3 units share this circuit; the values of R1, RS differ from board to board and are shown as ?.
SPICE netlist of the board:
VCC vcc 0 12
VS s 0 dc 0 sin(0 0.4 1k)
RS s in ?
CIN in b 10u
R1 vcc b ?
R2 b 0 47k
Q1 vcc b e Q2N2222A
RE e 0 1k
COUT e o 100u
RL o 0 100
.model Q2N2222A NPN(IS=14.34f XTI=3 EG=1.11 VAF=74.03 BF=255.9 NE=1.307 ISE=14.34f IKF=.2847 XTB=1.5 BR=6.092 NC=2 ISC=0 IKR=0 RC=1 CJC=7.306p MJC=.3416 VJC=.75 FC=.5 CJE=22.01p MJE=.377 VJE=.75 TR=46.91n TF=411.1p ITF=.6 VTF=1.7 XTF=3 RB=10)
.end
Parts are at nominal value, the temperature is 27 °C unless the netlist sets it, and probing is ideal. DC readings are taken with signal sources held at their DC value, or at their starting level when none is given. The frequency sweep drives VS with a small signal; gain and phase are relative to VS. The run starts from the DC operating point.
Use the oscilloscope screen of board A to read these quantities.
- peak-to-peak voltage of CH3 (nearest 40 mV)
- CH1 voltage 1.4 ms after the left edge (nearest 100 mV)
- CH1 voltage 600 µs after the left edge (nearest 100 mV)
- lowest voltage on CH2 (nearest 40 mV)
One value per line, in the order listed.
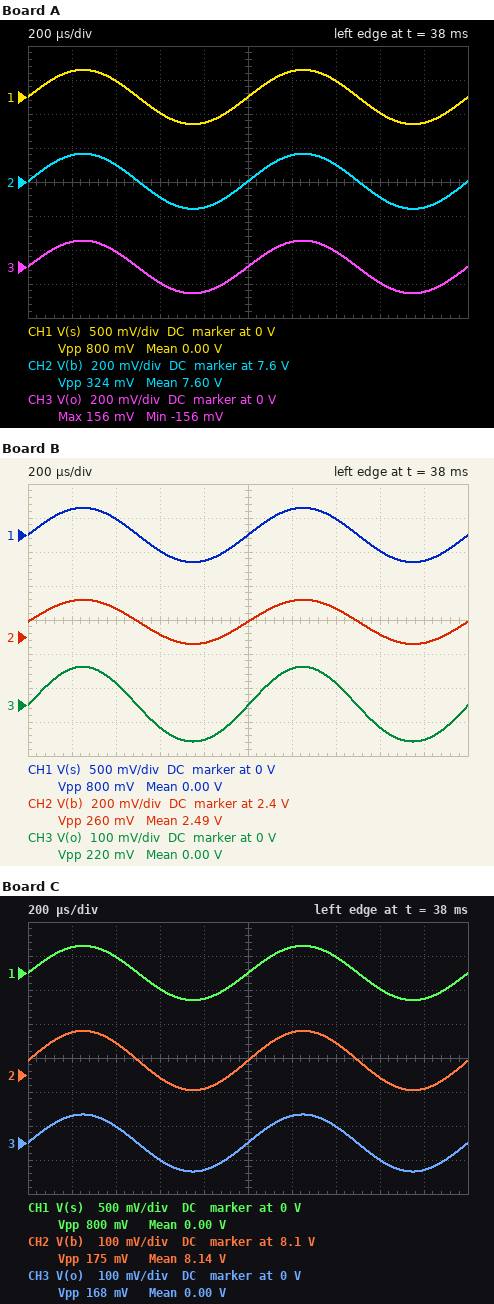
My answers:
320 mV
200 mV
-200 mV
7.44 V
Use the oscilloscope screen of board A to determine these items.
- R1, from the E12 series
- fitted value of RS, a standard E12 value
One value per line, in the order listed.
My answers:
22 kΩ
12 kΩ
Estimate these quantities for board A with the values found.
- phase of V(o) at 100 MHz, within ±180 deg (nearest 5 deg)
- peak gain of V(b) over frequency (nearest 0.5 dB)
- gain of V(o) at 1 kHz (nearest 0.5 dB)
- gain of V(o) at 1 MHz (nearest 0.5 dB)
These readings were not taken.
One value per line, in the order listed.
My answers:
-75 deg
-6.0 dB
-8.0 dB
-8.5 dB
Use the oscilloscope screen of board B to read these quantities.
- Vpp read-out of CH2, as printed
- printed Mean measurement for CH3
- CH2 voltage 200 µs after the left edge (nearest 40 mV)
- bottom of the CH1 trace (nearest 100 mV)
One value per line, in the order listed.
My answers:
260 mV
0.00 V
2.60 V
-400 mV
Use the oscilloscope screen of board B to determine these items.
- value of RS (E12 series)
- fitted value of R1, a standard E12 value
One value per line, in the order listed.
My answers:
27 kΩ
150 kΩ
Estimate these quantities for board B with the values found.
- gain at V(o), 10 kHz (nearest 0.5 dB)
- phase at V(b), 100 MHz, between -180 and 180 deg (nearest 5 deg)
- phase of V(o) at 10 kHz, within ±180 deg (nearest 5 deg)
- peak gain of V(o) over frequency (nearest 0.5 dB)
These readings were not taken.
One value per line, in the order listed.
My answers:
-11.0 dB
-65 deg
0 deg
-11.0 dB
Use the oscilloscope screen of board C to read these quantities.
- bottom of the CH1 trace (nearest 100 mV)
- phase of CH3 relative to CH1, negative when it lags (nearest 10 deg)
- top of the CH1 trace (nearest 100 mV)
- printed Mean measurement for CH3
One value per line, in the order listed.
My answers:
-400 mV
0 deg
400 mV
0.00 V
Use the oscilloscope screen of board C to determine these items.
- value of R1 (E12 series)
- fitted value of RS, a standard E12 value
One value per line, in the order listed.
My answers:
18 kΩ
27 kΩ
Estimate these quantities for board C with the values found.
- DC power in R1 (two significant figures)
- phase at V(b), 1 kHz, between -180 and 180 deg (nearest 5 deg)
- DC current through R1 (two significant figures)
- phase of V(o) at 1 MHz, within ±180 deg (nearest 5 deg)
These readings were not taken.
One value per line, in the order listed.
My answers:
830 µW
0 deg
210 µA
-20 deg
